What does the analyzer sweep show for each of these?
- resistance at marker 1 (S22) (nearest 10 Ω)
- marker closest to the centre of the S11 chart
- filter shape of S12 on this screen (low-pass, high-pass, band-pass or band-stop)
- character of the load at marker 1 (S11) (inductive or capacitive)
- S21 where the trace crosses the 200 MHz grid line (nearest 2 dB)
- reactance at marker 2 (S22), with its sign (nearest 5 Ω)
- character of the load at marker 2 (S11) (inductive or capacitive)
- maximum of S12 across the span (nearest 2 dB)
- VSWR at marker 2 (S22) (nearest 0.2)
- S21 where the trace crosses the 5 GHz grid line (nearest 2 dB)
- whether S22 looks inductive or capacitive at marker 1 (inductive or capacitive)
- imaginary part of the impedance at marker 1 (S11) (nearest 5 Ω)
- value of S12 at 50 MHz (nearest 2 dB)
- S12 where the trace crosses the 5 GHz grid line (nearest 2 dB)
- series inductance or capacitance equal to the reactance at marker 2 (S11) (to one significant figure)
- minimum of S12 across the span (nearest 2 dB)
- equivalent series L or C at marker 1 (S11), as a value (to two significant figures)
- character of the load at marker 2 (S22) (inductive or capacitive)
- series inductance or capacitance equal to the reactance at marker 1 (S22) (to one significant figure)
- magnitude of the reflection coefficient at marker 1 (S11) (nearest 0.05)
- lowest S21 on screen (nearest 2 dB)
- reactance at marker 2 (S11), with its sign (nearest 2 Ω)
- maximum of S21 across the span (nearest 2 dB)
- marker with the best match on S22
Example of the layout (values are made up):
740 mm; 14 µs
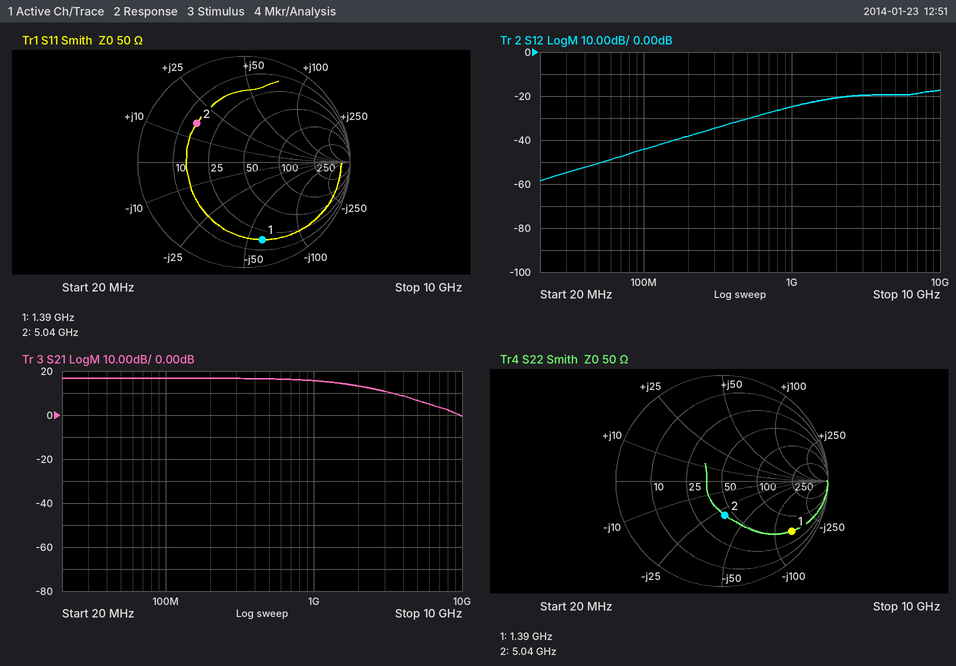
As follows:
50 Ω; marker 2; high-pass; capacitive; 16 dB; -30 Ω; inductive; -18 dB; 2.0; 6 dB; capacitive; -60 Ω; -50 dB; -20 dB; 500 pH; -58 dB; 1.9 pF; capacitive; 800 fF; 0.75; 0 dB; +16 Ω; 16 dB; marker 2
